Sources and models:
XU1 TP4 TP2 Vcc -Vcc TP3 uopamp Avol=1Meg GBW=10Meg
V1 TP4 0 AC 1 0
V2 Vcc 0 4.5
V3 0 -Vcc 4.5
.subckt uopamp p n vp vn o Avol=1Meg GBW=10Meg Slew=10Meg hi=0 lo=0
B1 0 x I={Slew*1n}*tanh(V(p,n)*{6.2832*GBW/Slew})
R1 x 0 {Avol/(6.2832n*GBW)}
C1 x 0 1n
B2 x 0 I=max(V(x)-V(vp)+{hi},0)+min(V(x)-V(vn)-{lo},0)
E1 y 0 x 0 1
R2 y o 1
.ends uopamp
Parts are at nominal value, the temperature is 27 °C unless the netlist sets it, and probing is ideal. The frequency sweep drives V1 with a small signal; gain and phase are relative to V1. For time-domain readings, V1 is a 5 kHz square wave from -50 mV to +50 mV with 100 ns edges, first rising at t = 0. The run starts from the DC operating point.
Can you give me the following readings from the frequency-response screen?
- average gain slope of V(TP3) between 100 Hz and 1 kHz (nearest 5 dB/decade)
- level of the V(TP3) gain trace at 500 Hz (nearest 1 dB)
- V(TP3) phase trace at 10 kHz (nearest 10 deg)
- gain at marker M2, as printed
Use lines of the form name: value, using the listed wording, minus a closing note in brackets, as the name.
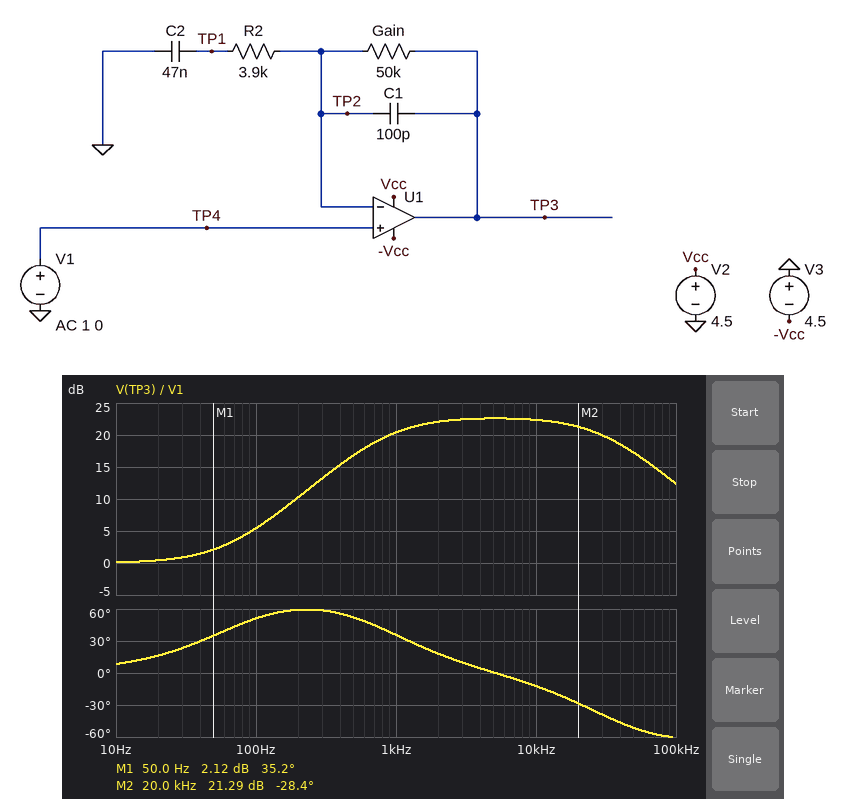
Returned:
average gain slope of V(TP3) between 100 Hz and 1 kHz: 15 dB/decade
level of the V(TP3) gain trace at 500 Hz: 17 dB
V(TP3) phase trace at 10 kHz: -10 deg
gain at marker M2, as printed: 21.29 dB
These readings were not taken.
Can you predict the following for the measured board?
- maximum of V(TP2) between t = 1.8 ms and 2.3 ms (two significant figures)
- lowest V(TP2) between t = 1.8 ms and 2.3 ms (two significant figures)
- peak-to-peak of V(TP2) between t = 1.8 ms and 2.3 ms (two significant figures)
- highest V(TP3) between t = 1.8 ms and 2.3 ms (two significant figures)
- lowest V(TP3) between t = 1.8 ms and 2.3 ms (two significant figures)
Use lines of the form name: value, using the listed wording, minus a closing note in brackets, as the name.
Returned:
maximum of V(TP2) between t = 1.8 ms and 2.3 ms: 50 mV
lowest V(TP2) between t = 1.8 ms and 2.3 ms: -50 mV
peak-to-peak of V(TP2) between t = 1.8 ms and 2.3 ms: 100 mV
highest V(TP3) between t = 1.8 ms and 2.3 ms: 770 mV
lowest V(TP3) between t = 1.8 ms and 2.3 ms: -770 mV
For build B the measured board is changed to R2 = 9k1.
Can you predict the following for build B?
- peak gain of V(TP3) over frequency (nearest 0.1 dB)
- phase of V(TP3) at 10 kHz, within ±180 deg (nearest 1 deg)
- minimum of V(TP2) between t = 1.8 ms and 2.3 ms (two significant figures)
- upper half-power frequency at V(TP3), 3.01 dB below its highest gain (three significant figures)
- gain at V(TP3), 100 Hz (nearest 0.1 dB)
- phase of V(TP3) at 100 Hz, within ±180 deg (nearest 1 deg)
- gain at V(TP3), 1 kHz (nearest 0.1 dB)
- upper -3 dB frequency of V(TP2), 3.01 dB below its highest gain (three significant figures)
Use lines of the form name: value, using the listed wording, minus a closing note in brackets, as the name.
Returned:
peak gain of V(TP3) over frequency: 16.2 dB
phase of V(TP3) at 10 kHz, within ±180 deg: -13 deg
minimum of V(TP2) between t = 1.8 ms and 2.3 ms: -50 mV
upper half-power frequency at V(TP3), 3.01 dB below its highest gain: 32.8 kHz
gain at V(TP3), 100 Hz: 5.8 dB
phase of V(TP3) at 100 Hz, within ±180 deg: 45 deg
gain at V(TP3), 1 kHz: 15.7 dB
upper -3 dB frequency of V(TP2), 3.01 dB below its highest gain: 9.82 MHz
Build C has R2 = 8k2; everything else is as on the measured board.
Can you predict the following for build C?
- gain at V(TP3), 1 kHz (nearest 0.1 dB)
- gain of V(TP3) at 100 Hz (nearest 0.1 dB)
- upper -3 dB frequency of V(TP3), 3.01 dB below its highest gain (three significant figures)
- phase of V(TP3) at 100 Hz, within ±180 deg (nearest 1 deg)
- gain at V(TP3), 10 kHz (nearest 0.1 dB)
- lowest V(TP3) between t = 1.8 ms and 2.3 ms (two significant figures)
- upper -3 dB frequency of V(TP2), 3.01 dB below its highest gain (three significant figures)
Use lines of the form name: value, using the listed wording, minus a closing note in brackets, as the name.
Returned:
gain at V(TP3), 1 kHz: 16.4 dB
gain of V(TP3) at 100 Hz: 5.7 dB
upper -3 dB frequency of V(TP3), 3.01 dB below its highest gain: 32.7 kHz
phase of V(TP3) at 100 Hz, within ±180 deg: 46 deg
gain at V(TP3), 10 kHz: 16.6 dB
lowest V(TP3) between t = 1.8 ms and 2.3 ms: -370 mV
upper -3 dB frequency of V(TP2), 3.01 dB below its highest gain: 9.80 MHz
